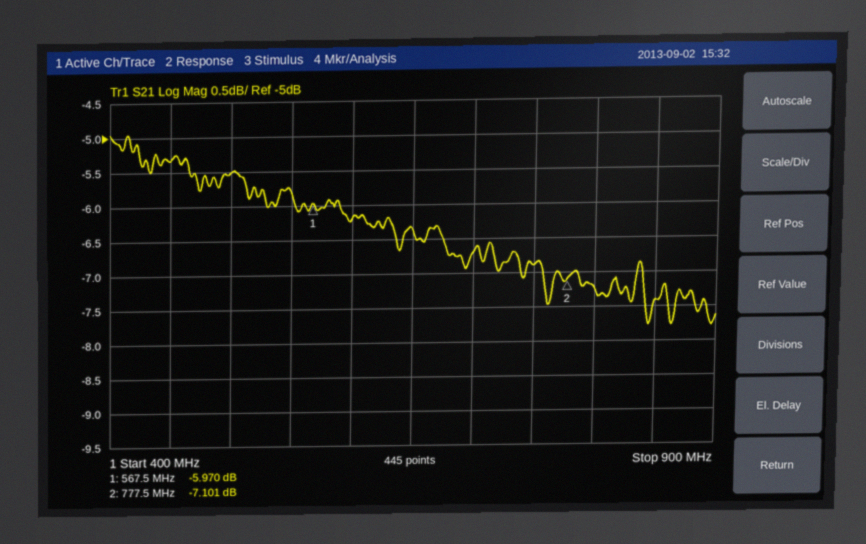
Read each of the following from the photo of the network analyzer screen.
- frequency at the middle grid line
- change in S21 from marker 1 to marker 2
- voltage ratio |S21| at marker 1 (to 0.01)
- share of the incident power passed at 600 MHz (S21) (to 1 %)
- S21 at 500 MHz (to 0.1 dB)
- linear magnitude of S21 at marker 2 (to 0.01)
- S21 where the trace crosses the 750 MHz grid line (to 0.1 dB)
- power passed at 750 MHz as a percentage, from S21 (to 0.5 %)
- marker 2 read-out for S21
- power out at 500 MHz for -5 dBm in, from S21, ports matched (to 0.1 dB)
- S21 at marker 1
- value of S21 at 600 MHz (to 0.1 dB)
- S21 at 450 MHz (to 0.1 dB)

650 MHz
-1.131 dB
0.50
24 %
-5.5 dB
0.44
-6.9 dB
20.5 %
-7.101 dB
-10.5 dBm
-5.970 dB
-6.2 dB
-5.3 dB
